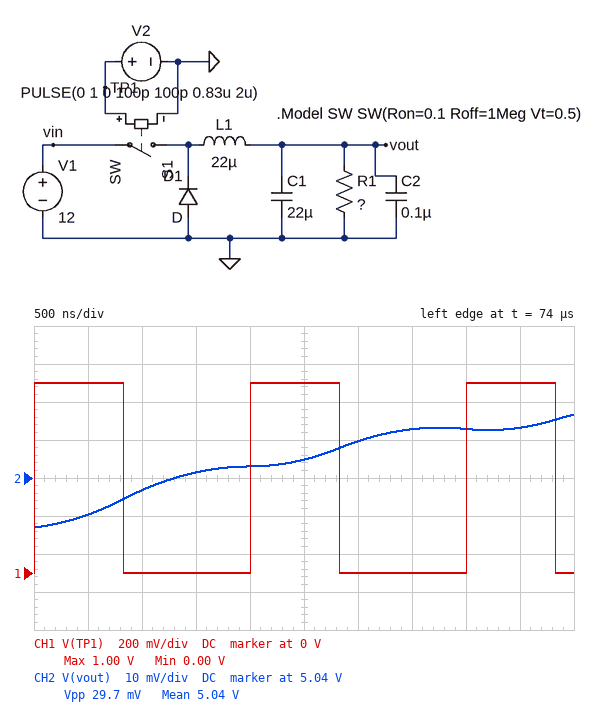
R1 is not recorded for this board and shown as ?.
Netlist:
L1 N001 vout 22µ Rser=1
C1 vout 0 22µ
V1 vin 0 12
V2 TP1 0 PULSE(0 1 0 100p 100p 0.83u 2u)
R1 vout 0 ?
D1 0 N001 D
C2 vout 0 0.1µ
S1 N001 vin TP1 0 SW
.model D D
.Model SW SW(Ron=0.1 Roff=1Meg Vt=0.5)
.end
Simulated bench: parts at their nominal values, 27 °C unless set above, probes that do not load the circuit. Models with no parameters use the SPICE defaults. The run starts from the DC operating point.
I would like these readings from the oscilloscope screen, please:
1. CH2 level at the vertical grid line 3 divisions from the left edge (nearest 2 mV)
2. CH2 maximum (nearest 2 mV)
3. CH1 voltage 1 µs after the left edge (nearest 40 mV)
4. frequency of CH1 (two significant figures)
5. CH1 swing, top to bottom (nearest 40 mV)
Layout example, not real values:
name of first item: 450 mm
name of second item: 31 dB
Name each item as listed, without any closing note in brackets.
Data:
CH2 level at the vertical grid line 3 divisions from the left edge: 5.042 V
CH2 maximum: 5.056 V
CH1 voltage 1 µs after the left edge: 0 V
frequency of CH1: 500 kHz
CH1 swing, top to bottom: 1.00 V
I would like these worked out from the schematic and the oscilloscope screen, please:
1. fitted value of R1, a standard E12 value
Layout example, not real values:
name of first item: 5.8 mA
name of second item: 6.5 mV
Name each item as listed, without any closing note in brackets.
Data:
fitted value of R1, a standard E12 value: 68 Ω
